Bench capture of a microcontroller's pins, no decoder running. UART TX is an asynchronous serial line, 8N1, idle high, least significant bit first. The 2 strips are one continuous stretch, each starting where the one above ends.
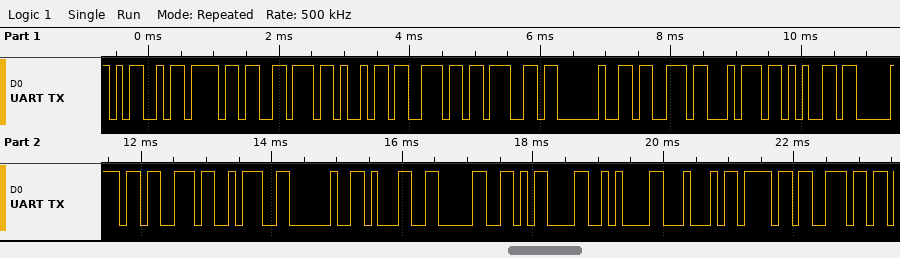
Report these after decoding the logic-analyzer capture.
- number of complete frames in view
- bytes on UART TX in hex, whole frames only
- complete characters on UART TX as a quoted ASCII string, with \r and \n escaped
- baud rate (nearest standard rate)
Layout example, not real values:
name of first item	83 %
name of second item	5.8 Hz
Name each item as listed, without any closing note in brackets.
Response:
number of complete frames in view	21
bytes on UART TX in hex, whole frames only	0x4D 0x6F 0x76 0x69 0x6E 0x67 0x20 0x73 0x74 0x65 0x70 0x73 0x3A 0x20 0x31 0x30 0x0D 0x0A 0x44 0x6F 0x6E
complete characters on UART TX as a quoted ASCII string, with \r and \n escaped	"Moving steps: 10\r\nDon"
baud rate	9600 baud
